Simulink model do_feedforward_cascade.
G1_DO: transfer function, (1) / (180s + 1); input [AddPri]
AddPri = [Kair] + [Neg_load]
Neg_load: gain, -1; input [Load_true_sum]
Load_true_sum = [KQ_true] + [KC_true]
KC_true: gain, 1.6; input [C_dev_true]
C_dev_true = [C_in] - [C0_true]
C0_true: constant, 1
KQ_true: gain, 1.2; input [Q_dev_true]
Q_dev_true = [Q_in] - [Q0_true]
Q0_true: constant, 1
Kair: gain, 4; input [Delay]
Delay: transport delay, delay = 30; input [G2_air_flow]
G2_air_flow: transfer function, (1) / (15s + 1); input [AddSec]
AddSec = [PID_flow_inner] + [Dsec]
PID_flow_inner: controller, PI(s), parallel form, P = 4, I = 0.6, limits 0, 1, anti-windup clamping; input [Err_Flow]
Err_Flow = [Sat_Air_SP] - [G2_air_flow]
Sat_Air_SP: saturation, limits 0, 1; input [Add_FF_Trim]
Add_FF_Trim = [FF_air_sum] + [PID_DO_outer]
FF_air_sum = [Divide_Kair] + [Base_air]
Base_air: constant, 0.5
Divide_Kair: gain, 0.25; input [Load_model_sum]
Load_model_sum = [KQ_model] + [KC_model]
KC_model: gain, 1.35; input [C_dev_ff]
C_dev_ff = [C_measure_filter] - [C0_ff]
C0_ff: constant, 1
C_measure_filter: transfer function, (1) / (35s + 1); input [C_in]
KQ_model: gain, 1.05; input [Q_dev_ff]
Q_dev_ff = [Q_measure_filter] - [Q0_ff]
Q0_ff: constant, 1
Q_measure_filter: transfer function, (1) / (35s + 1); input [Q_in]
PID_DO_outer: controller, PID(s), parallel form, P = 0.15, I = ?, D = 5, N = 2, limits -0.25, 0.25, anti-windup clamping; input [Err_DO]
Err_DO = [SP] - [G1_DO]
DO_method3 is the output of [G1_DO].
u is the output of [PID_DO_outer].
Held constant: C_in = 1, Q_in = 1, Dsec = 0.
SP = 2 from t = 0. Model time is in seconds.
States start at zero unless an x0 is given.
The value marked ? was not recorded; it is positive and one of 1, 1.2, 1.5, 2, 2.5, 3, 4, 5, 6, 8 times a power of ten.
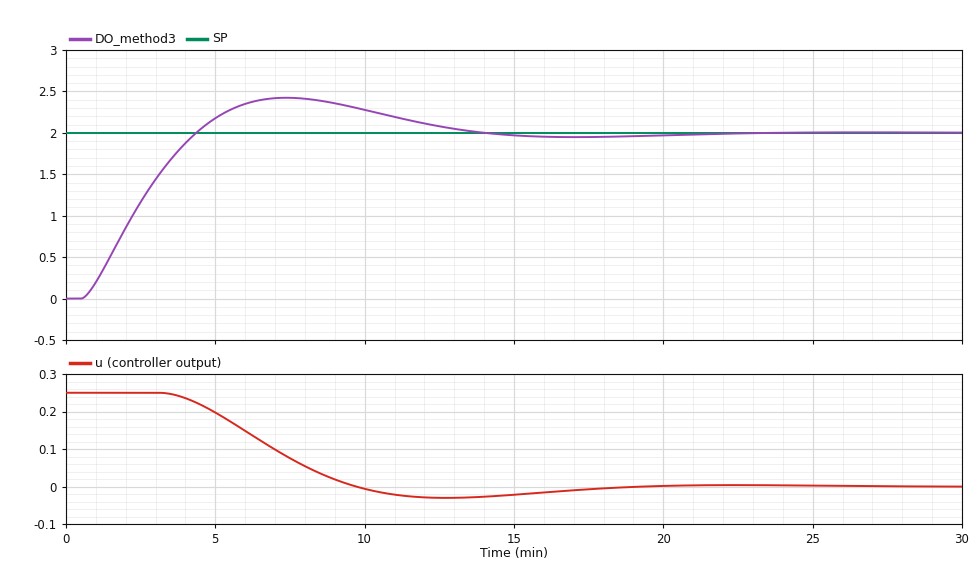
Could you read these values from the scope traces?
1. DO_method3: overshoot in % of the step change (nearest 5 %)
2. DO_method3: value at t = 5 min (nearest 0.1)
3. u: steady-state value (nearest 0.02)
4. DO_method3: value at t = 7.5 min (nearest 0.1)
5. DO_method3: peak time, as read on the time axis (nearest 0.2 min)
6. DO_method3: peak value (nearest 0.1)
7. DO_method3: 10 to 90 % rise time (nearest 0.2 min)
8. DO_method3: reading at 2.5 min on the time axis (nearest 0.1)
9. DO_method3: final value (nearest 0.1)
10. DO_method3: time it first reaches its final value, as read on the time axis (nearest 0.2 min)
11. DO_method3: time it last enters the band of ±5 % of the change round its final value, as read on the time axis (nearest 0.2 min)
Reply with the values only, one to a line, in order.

20 %
2.2
0.00
2.4
7.4 min
2.4
2.8 min
1.2
2.0
4.4 min
12.2 min
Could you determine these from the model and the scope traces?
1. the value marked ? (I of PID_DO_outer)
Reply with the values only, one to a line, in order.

0.002
